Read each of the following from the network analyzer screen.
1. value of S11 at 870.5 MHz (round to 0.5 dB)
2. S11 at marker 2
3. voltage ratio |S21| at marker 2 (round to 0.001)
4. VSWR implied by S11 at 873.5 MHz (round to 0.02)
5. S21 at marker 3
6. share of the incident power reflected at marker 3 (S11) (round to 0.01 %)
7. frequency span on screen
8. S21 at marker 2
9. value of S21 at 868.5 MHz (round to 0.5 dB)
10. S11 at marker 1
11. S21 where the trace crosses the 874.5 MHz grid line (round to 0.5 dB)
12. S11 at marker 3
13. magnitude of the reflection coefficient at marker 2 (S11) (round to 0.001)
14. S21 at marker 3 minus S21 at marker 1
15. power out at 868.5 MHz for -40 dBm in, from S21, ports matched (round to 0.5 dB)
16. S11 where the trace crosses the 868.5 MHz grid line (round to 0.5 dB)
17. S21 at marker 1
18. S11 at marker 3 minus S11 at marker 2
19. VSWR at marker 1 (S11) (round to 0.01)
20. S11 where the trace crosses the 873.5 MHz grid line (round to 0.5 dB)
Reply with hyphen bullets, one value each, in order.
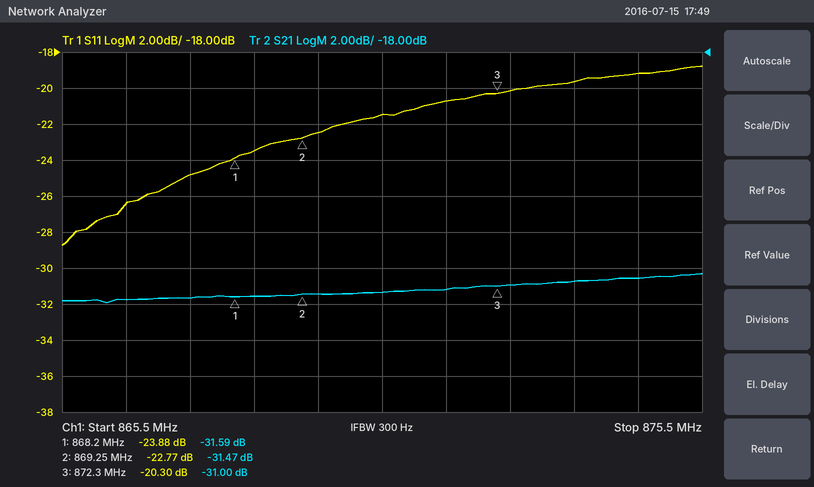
- -21.5 dB
- -22.77 dB
- 0.027
- 1.24
- -31.00 dB
- 0.93 %
- 10 MHz
- -31.47 dB
- -31.5 dB
- -23.88 dB
- -30.5 dB
- -20.30 dB
- 0.073
- 0.59 dB
- -71.5 dBm
- -23.5 dB
- -31.59 dB
- 2.47 dB
- 1.14
- -19.5 dB
